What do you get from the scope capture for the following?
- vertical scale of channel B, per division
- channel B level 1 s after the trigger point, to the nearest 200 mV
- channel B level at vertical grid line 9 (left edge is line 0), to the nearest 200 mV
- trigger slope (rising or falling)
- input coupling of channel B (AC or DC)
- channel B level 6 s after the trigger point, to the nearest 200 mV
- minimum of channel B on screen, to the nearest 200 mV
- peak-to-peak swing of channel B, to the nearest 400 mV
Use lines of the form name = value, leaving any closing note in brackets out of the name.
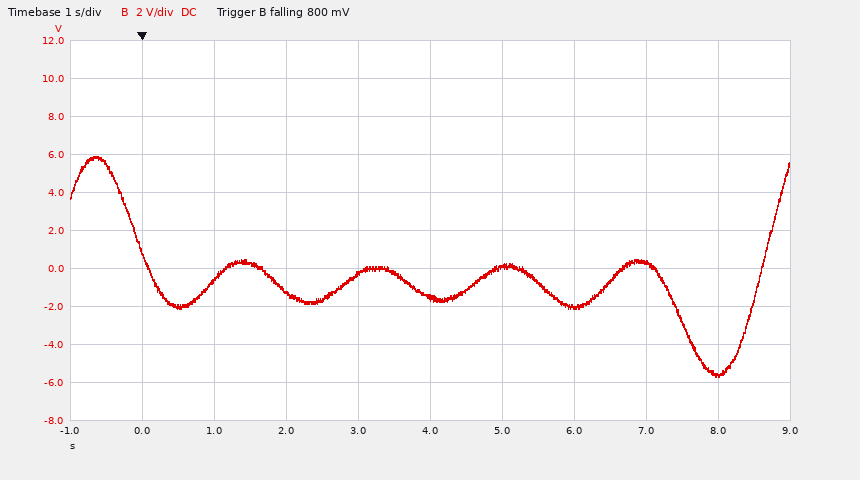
vertical scale of channel B, per division = 2 V
channel B level 1 s after the trigger point, to the nearest 200 mV = -600 mV
channel B level at vertical grid line 9 (left edge is line 0), to the nearest 200 mV = -5.6 V
trigger slope = falling
input coupling of channel B = DC
channel B level 6 s after the trigger point, to the nearest 200 mV = -2.0 V
minimum of channel B on screen, to the nearest 200 mV = -5.6 V
peak-to-peak swing of channel B, to the nearest 400 mV = 11.6 V
